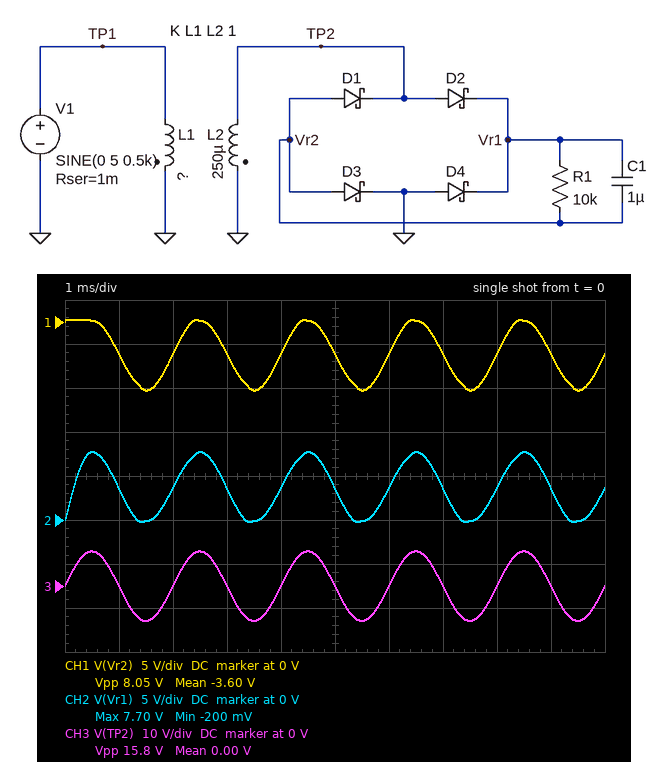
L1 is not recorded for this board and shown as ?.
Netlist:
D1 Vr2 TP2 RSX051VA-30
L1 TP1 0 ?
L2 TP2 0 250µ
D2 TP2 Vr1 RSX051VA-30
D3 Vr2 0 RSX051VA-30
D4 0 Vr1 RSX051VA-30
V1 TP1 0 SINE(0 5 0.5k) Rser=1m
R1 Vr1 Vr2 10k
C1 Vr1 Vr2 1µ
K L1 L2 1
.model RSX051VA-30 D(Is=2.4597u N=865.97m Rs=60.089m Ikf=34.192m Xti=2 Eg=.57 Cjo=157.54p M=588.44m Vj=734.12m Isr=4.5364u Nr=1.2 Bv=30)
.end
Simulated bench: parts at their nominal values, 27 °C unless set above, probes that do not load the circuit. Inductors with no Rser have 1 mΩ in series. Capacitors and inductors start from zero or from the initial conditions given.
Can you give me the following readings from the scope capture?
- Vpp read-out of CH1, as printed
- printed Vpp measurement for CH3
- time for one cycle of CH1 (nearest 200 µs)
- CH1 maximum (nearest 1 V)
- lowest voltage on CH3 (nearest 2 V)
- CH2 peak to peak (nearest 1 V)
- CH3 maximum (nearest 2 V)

8.05 V
15.8 V
2.0 ms
0 V
-8 V
8 V
8 V
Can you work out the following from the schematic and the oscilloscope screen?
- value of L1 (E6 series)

100 µH
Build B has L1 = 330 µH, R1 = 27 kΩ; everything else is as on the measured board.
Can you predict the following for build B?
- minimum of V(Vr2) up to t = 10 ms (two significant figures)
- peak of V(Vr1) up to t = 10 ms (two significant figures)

-4.2 V
4.2 V
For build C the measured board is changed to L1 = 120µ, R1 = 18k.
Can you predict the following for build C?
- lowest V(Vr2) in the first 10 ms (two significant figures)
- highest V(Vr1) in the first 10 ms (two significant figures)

-7.1 V
7.0 V
